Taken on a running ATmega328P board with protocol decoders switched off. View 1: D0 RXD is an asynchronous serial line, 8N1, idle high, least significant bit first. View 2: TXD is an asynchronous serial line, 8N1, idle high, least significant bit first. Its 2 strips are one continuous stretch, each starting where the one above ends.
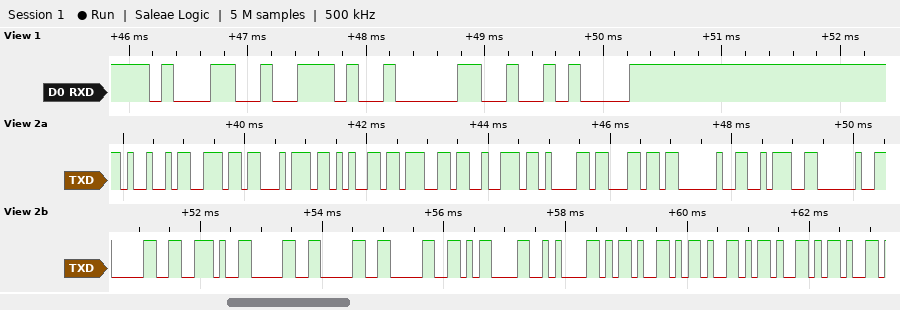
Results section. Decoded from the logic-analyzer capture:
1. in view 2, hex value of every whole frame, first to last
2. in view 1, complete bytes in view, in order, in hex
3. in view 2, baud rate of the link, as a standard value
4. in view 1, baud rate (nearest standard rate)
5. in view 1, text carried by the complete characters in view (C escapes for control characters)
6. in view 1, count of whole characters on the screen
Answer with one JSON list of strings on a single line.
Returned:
["49 6E 74 65 67 72 61 6C 20 3A 20 30 2E 30 30 30 0D 0A 2D 2D 2D 2D", "31 2E 30 0A", "9600 baud", "9600 baud", "\"1.0\\n\"", "4"]
